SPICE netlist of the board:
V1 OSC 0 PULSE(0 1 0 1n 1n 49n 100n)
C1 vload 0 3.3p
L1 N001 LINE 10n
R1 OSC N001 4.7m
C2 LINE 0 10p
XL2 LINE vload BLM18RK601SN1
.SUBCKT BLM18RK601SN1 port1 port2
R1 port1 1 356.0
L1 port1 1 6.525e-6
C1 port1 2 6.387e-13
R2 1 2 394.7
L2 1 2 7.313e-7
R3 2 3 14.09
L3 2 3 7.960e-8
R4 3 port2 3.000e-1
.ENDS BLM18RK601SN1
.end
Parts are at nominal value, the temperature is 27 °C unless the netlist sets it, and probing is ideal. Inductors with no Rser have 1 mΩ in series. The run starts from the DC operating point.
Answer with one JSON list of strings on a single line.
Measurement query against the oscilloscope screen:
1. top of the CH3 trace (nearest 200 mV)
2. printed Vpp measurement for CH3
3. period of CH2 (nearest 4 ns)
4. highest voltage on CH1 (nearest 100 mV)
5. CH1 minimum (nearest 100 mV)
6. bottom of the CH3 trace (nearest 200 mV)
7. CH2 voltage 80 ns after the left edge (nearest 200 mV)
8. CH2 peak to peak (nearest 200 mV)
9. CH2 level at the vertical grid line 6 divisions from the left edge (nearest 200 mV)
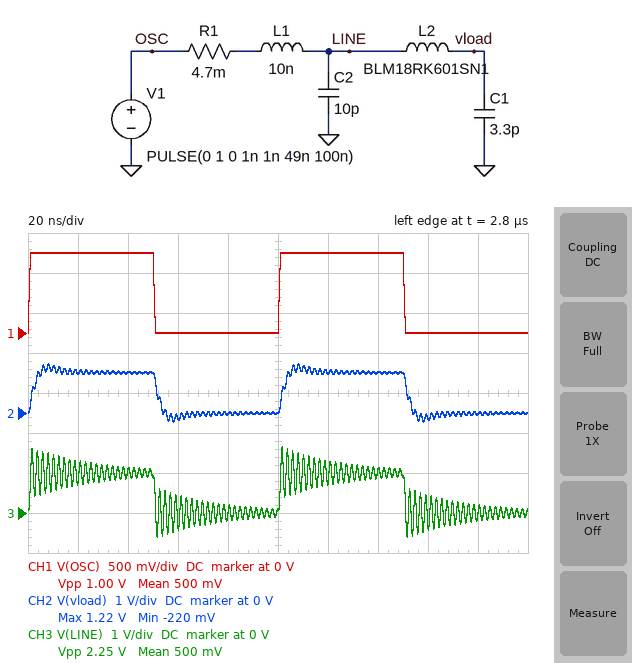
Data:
["1.6 V", "2.25 V", "100 ns", "1.0 V", "0 V", "-600 mV", "0 V", "1.4 V", "1.0 V"]
